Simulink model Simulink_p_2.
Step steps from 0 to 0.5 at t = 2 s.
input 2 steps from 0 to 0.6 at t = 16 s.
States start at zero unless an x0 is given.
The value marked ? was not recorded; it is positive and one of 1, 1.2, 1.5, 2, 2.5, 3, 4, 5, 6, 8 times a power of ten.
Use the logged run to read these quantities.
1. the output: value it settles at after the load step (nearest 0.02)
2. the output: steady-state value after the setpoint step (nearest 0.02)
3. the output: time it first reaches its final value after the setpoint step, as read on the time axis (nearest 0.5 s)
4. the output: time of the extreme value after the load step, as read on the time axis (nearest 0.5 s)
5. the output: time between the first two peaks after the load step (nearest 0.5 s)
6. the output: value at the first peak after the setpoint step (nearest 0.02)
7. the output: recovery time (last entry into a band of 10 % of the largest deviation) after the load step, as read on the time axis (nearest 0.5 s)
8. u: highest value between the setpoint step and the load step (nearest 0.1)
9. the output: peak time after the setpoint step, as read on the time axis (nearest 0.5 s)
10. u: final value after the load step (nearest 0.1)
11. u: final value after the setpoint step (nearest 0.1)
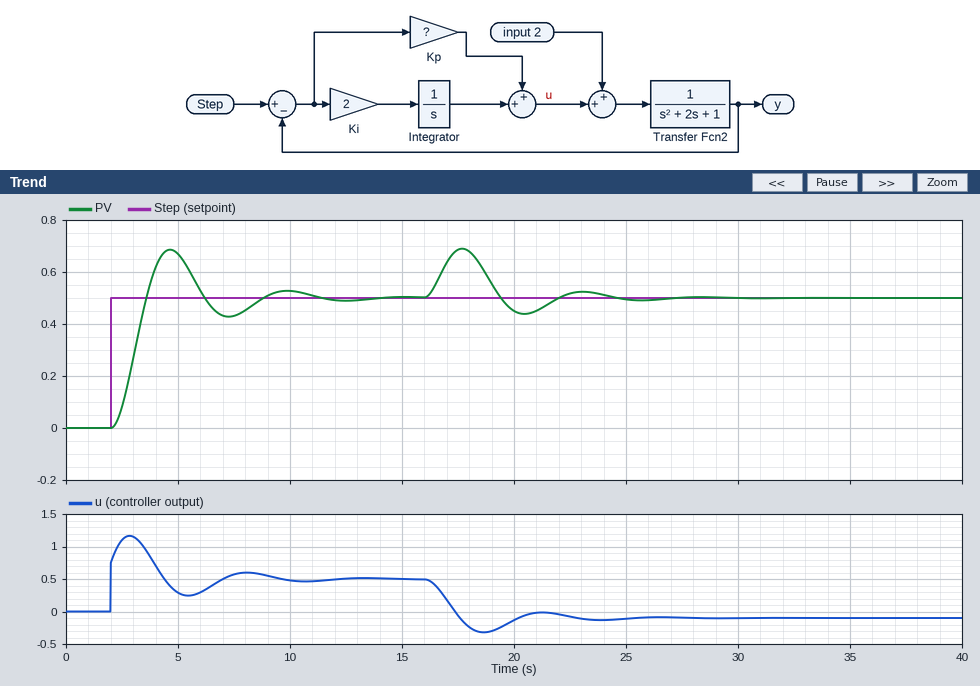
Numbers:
0.50
0.50
3.5 s
17.5 s
5.5 s
0.68
23.5 s
1.2
4.5 s
-0.1
0.5
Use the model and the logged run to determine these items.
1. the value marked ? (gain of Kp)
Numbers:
1.5
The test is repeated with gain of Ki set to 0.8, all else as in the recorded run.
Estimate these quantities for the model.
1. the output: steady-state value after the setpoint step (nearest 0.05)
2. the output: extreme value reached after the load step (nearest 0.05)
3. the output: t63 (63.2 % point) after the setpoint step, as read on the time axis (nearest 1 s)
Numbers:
0.50
0.70
3 s
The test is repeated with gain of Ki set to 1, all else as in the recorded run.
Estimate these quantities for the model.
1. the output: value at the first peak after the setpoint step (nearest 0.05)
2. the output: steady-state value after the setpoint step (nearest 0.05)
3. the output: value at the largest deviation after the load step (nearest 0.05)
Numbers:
0.55
0.50
0.70
